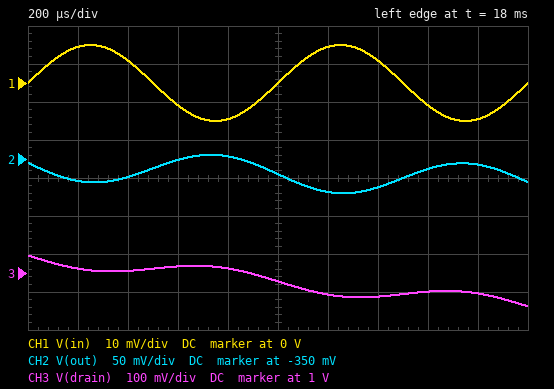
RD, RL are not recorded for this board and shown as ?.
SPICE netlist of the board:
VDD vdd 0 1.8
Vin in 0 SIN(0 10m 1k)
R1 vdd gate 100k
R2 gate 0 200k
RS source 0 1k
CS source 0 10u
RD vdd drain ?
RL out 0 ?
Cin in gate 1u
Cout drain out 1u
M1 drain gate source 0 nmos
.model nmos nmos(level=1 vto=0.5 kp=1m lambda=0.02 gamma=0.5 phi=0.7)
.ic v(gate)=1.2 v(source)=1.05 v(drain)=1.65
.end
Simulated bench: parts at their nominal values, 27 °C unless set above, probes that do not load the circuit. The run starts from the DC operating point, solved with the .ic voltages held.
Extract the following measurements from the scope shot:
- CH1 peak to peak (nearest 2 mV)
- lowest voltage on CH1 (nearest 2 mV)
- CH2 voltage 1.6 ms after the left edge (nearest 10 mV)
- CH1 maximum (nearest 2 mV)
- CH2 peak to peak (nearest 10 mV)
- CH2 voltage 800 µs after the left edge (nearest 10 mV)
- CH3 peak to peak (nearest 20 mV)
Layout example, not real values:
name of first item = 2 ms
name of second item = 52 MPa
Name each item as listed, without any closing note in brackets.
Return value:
CH1 peak to peak = 20 mV
lowest voltage on CH1 = -10 mV
CH2 voltage 1.6 ms after the left edge = -360 mV
CH1 maximum = 10 mV
CH2 peak to peak = 50 mV
CH2 voltage 800 µs after the left edge = -350 mV
CH3 peak to peak = 140 mV
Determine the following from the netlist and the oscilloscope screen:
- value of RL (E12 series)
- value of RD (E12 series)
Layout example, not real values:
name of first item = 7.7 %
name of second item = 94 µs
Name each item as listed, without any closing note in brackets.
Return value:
value of RL = 6.8 kΩ
value of RD = 18 kΩ
